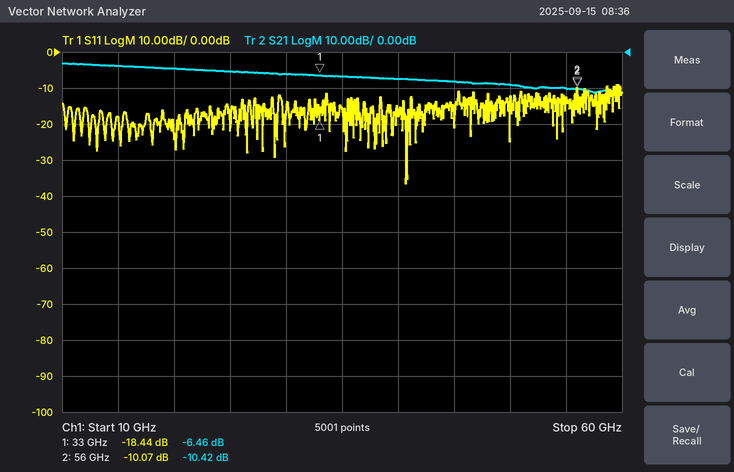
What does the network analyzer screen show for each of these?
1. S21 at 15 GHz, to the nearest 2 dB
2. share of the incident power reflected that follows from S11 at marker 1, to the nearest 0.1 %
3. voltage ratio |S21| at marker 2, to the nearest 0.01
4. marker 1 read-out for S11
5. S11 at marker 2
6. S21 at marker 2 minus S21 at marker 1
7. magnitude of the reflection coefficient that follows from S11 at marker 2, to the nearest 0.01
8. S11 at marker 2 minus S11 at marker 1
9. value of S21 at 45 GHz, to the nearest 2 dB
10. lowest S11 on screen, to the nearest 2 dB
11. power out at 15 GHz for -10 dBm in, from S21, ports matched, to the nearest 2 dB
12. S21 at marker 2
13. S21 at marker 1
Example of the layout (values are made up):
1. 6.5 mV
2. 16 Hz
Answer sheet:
1. -4 dB
2. 1.4 %
3. 0.30
4. -18.44 dB
5. -10.07 dB
6. -3.96 dB
7. 0.31
8. 8.37 dB
9. -8 dB
10. -36 dB
11. -14 dBm
12. -10.42 dB
13. -6.46 dB
